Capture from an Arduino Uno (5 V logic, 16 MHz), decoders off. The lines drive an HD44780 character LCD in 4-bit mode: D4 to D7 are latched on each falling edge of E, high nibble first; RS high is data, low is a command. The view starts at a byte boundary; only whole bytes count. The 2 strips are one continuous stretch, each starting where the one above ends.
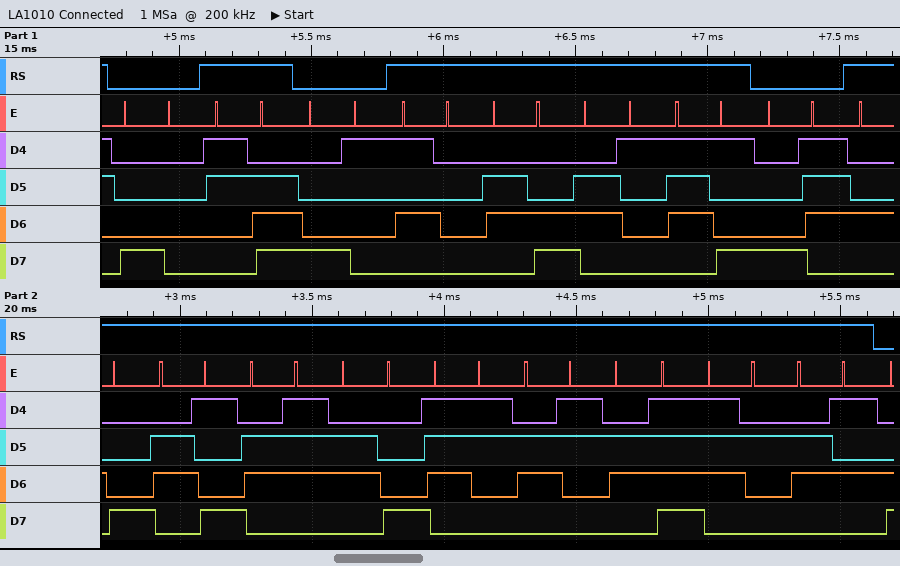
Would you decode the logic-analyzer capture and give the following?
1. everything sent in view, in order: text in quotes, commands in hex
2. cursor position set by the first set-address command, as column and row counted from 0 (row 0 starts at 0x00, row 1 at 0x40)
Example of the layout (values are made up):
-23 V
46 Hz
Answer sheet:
0x80 ">" 0x81 "Play" 0x87 "Highscore"
column 0, row 0
